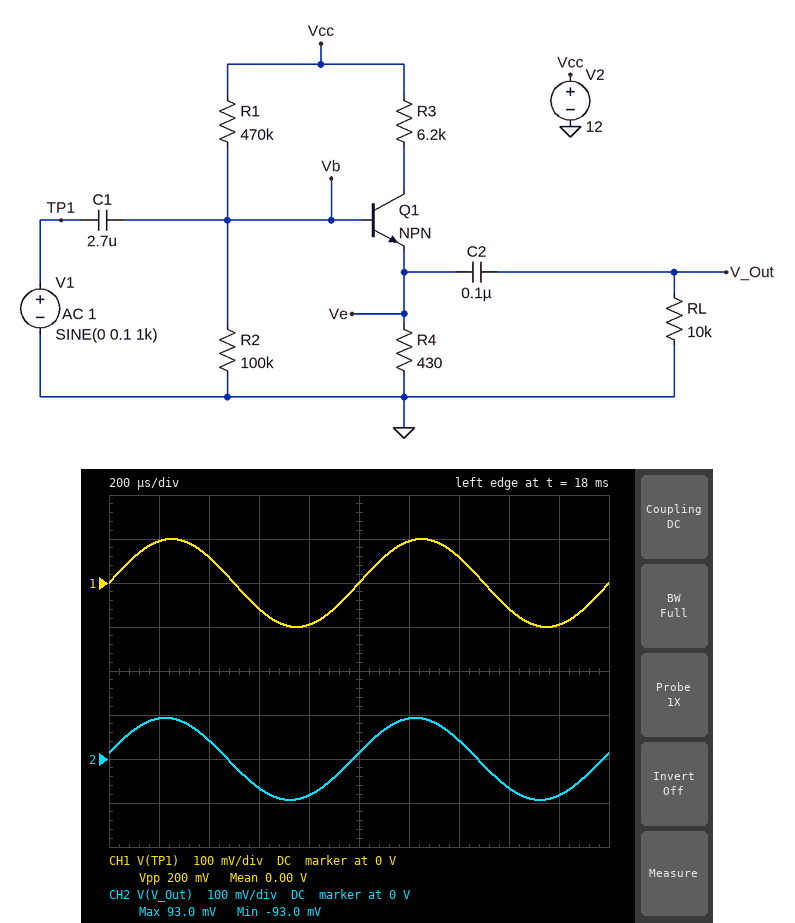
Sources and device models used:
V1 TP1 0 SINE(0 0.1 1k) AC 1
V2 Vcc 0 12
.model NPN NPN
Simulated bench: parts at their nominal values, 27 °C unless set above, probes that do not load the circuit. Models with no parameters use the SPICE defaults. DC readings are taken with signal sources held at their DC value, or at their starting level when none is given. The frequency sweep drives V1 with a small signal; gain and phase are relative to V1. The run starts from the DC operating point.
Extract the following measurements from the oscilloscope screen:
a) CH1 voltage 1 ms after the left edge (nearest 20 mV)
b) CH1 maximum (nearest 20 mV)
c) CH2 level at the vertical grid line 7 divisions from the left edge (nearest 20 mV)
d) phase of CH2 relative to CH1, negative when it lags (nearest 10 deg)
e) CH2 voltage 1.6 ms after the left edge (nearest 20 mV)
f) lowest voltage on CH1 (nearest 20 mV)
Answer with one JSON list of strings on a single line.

["0 V", "100 mV", "40 mV", "10 deg", "-60 mV", "-100 mV"]
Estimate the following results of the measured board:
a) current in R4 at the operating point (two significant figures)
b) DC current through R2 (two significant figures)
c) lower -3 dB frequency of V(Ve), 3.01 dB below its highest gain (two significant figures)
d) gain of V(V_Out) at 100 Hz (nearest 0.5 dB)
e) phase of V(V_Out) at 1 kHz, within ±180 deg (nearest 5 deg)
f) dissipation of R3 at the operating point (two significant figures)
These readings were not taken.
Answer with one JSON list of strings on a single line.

["1.1 mA", "12 µA", "2.0 Hz", "-6.0 dB", "10 deg", "6.9 mW"]
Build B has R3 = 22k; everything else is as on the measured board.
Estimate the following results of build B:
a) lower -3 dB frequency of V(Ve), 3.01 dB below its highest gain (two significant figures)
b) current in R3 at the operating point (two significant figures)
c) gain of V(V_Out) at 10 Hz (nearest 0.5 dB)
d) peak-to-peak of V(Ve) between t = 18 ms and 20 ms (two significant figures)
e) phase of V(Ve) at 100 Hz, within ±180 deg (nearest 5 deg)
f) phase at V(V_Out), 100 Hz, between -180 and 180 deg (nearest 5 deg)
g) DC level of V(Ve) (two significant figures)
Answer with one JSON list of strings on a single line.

["100 Hz", "530 µA", "-46.0 dB", "170 mV", "45 deg", "105 deg", "230 mV"]
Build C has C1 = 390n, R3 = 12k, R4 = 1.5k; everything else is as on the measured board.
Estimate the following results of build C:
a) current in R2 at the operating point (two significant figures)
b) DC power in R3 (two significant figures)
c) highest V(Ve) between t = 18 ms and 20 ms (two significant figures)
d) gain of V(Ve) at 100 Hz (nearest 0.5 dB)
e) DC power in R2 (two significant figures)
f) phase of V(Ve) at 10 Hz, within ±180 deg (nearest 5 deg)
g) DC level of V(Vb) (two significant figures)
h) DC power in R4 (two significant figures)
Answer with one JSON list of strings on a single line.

["16 µA", "4.0 mW", "970 mV", "-0.5 dB", "27 µW", "35 deg", "1.6 V", "510 µW"]
